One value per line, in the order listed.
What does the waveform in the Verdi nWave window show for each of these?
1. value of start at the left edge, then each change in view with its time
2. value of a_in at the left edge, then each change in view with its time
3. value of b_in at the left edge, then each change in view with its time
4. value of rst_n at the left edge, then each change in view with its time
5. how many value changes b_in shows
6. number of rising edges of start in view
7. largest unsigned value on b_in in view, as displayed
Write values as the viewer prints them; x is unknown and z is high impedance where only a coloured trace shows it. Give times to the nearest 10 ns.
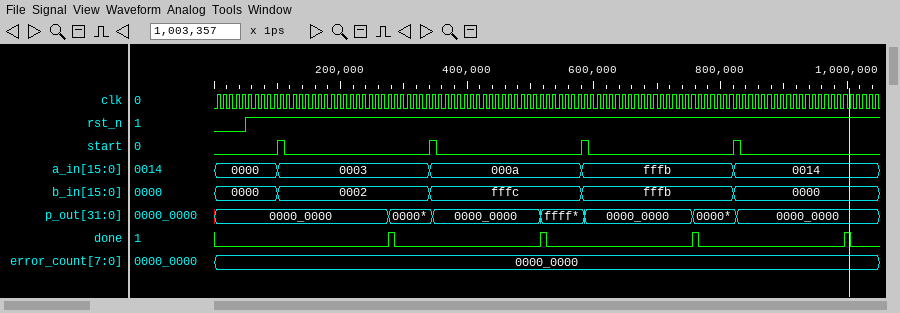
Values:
0, 1 at 100 ns, 0 at 110 ns, 1 at 340 ns, 0 at 350 ns, 1 at 580 ns, 0 at 590 ns, 1 at 820 ns, 0 at 830 ns
0000, 0003 at 100 ns, 000a at 340 ns, fffb at 580 ns, 0014 at 820 ns
0000, 0002 at 100 ns, fffc at 340 ns, fffb at 580 ns, 0000 at 820 ns
0, 1 at 50 ns
4
4
fffc
